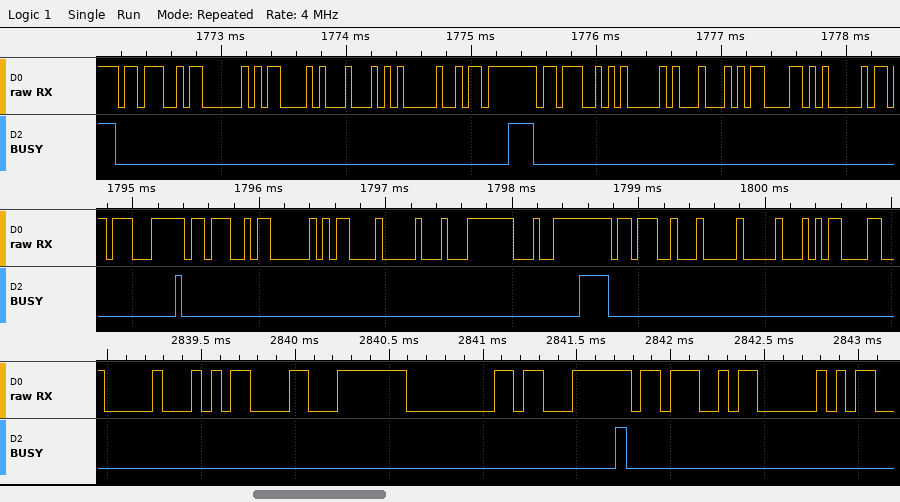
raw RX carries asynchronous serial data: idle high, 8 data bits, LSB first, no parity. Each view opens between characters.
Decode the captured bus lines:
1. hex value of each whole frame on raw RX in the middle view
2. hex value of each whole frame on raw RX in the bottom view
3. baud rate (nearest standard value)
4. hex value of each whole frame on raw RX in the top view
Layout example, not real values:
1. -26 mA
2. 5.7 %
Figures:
1. C7, 3B, 03, 0D, 10, FC, E4, 3B, 04, 10, 0D
2. 10, 0D, FC, 00, E3, 3B, 03
3. 19200 baud
4. 3B, 03, 0D, 11, 05, DA, 3B, 05, 11, 0D, 05
